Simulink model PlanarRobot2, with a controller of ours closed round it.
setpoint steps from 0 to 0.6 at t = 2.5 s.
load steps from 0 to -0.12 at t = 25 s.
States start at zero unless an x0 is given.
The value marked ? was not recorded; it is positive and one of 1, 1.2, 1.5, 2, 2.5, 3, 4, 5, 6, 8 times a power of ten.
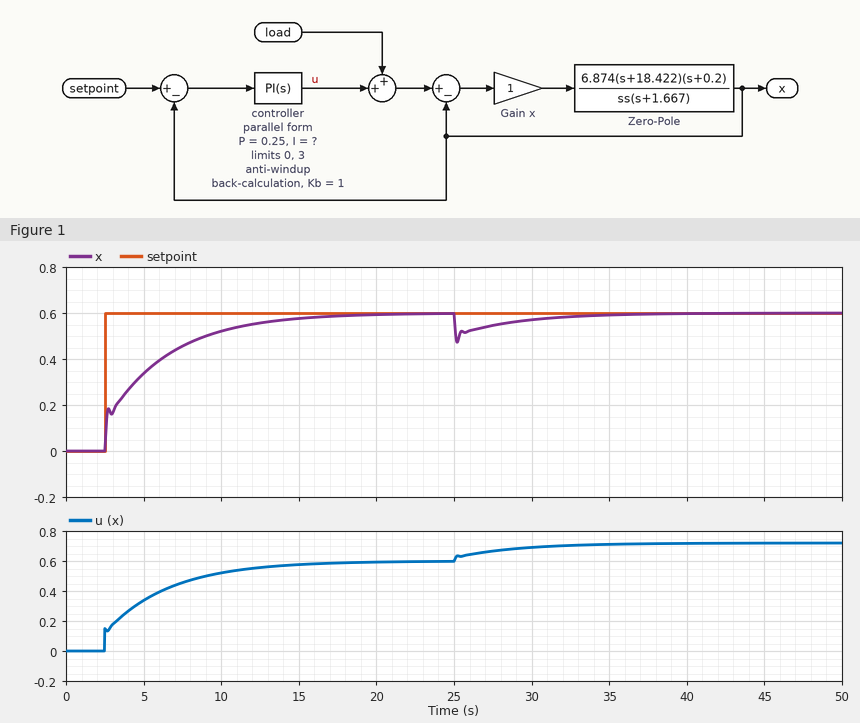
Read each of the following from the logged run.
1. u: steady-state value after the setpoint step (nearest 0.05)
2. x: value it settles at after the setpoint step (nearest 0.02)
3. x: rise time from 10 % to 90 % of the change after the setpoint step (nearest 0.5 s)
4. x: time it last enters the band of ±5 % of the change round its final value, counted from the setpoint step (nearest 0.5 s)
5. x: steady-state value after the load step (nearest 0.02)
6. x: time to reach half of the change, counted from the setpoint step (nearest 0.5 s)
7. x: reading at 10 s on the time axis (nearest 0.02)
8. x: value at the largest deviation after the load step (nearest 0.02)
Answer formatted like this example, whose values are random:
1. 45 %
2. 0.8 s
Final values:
1. 0.60
2. 0.60
3. 8.5 s
4. 11.5 s
5. 0.60
6. 2.0 s
7. 0.52
8. 0.48
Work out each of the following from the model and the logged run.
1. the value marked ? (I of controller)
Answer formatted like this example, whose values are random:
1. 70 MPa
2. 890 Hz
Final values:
1. 0.3
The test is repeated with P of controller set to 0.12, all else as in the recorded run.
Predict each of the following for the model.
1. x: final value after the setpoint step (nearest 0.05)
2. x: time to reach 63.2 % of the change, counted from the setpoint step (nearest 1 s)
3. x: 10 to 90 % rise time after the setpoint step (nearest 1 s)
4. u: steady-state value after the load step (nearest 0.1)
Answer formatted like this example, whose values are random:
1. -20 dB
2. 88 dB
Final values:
1. 0.60
2. 3 s
3. 8 s
4. 0.7
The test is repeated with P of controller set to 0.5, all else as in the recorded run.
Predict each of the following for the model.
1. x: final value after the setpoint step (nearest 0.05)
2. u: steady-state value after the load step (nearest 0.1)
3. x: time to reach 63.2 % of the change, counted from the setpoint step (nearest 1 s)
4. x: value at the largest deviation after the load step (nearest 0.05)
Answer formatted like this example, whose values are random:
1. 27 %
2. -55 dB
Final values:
1. 0.60
2. 0.7
3. 3 s
4. 0.50
